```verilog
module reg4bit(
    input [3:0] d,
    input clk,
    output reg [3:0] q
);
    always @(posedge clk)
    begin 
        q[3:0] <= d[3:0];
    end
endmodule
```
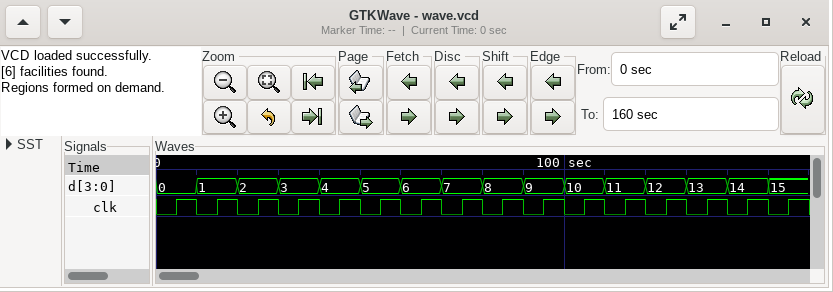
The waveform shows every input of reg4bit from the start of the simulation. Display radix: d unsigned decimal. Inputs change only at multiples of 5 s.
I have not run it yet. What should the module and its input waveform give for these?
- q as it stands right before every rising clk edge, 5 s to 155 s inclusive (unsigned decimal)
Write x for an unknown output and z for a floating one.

x, 0, 1, 2, 3, 4, 5, 6, 7, 8, 9, 10, 11, 12, 13, 14
